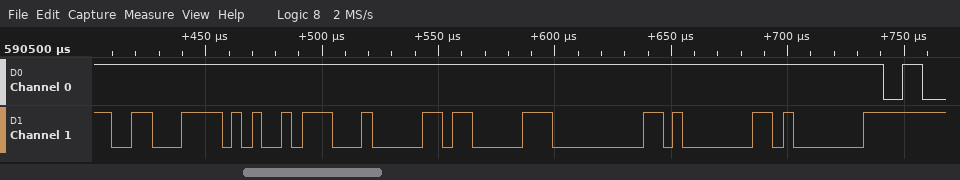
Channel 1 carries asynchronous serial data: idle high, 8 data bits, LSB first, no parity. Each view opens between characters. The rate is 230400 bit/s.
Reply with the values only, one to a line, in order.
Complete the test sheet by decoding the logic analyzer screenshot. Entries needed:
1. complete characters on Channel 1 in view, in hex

C6, A5, 04, 83, 00, 01, 01
